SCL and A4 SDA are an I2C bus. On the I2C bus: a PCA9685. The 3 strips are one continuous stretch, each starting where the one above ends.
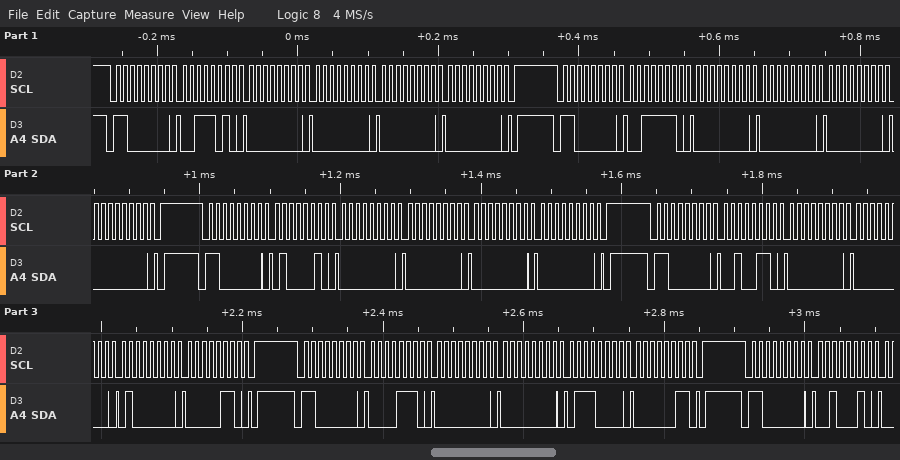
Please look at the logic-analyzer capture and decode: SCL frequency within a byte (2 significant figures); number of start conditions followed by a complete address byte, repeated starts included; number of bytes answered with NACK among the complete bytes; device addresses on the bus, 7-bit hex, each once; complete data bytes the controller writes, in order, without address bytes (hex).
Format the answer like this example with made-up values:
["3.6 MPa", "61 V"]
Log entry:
["100 kHz", "6", "0", "0x60", "3A 00 00 00 00 3E 00 00 00 00 42 00 00 00 00 26 00 00 40 06 0E 00 00 70 03 22"]
